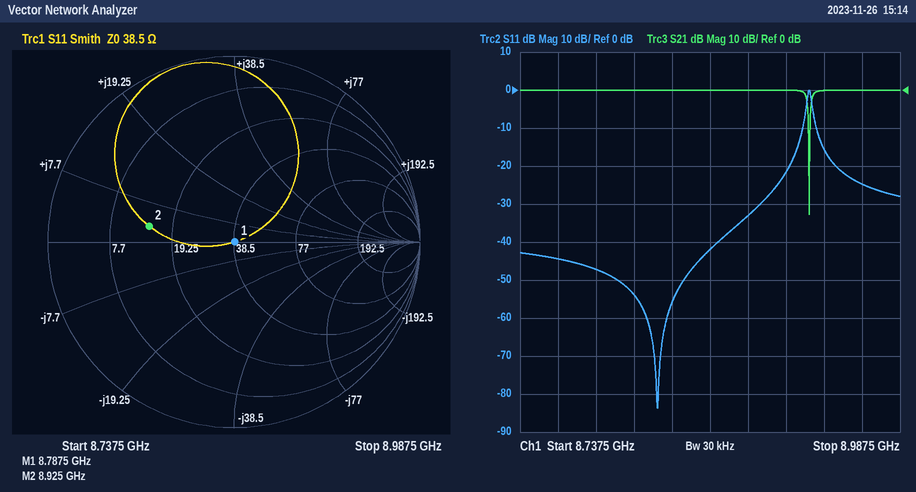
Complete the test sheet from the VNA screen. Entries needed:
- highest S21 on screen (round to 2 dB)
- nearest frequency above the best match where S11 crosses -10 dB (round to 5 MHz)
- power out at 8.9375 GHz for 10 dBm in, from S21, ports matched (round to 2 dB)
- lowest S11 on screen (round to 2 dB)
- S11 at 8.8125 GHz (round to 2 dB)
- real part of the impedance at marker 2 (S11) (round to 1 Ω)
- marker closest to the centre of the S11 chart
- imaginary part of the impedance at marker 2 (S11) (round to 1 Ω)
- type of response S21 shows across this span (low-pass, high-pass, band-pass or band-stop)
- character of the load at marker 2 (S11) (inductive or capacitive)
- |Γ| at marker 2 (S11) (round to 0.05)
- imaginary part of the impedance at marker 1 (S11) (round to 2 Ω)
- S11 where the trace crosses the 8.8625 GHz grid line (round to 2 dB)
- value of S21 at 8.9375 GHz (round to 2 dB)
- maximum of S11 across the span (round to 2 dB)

0 dB
8.925 GHz
10 dBm
-84 dB
-54 dB
14 Ω
marker 1
+3 Ω
band-stop
inductive
0.45
0 Ω
-42 dB
0 dB
0 dB
